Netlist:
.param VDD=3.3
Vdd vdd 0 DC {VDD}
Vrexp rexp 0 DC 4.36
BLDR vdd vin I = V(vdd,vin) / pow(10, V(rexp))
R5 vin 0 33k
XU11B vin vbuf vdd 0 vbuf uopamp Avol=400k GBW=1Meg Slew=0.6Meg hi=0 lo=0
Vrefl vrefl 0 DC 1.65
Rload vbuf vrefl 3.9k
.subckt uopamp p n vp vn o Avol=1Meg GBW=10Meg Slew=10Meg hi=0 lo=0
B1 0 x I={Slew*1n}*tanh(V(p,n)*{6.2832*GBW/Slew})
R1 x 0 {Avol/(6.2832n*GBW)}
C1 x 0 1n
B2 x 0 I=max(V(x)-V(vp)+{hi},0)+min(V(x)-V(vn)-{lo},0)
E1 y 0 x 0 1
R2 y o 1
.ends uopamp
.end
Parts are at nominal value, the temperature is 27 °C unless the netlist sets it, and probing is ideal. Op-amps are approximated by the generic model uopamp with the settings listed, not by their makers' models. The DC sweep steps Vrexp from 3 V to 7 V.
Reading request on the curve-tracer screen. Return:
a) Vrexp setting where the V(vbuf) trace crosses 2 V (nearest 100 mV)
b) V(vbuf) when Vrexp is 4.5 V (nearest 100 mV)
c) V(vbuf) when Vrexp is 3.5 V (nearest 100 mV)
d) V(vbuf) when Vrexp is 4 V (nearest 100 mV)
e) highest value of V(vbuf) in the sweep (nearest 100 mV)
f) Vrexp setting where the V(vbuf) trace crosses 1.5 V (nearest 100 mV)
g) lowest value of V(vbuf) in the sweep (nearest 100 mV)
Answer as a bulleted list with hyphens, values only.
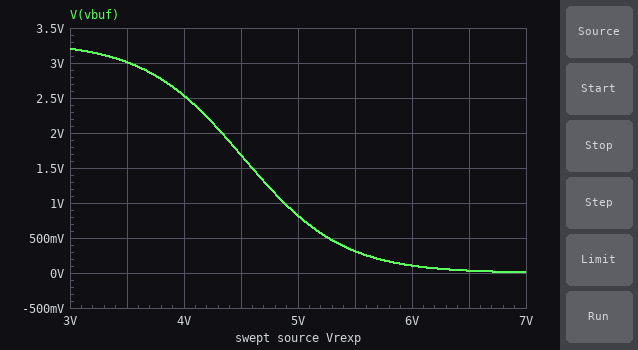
- 4.3 V
- 1.7 V
- 3.0 V
- 2.5 V
- 3.2 V
- 4.6 V
- 0 V
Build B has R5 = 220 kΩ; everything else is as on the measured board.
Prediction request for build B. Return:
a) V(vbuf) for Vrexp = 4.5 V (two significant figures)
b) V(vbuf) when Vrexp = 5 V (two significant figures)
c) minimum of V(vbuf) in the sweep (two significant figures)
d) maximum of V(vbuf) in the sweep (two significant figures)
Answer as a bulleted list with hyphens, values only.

- 2.9 V
- 2.3 V
- 71 mV
- 3.3 V
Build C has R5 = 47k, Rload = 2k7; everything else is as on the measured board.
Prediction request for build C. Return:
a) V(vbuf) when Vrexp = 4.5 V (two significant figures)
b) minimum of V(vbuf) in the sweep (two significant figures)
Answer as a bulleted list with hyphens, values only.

- 2.0 V
- 15 mV
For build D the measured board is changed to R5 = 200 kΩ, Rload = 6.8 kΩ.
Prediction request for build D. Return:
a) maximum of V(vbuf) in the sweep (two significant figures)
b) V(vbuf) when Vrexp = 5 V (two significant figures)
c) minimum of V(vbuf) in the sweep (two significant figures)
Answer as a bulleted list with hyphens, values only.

- 3.3 V
- 2.2 V
- 65 mV
